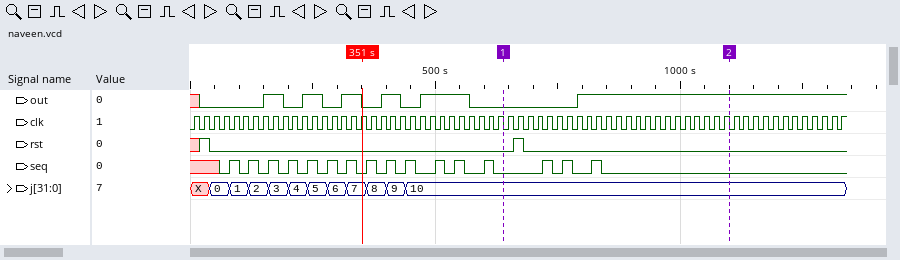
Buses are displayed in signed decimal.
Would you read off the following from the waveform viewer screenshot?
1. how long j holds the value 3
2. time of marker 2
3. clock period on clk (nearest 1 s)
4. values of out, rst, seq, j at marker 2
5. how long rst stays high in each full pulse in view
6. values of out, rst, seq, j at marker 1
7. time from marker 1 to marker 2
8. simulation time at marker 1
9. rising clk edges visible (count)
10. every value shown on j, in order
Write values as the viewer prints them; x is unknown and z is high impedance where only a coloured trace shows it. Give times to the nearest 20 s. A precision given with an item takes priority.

40 s
1100 s
20 s
out=1, rst=0, seq=0, j=10
20 s
out=0, rst=0, seq=0, j=10
460 s
640 s
67
X, 0, 1, 2, 3, 4, 5, 6, 7, 8, 9, 10
